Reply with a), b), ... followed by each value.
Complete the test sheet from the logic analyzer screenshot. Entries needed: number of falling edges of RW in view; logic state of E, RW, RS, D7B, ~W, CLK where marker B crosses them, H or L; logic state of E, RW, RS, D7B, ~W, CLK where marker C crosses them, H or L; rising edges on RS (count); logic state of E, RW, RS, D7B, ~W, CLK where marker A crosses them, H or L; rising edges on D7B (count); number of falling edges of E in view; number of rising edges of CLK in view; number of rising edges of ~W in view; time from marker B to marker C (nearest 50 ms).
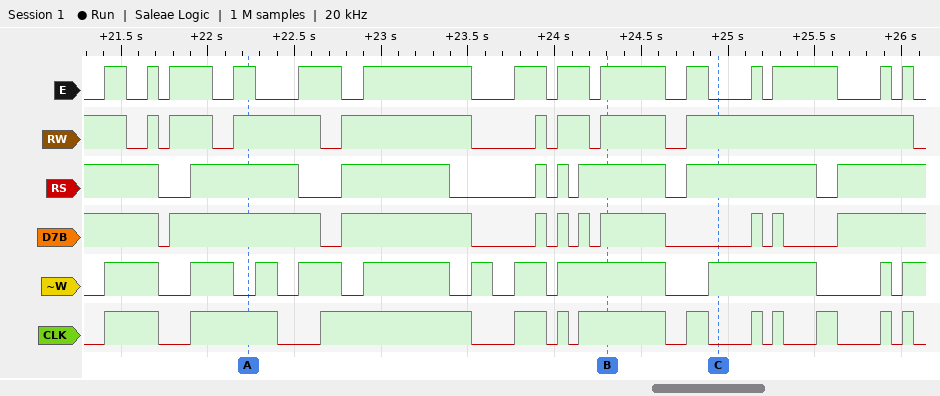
a) 9
b) E=H, RW=H, RS=H, D7B=H, ~W=H, CLK=H
c) E=L, RW=H, RS=H, D7B=L, ~W=H, CLK=L
d) 7
e) E=H, RW=H, RS=H, D7B=H, ~W=L, CLK=H
f) 9
g) 14
h) 12
i) 11
j) 650 ms
